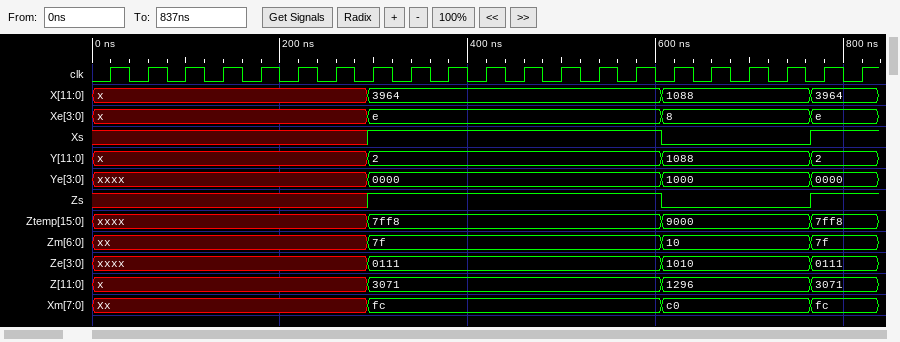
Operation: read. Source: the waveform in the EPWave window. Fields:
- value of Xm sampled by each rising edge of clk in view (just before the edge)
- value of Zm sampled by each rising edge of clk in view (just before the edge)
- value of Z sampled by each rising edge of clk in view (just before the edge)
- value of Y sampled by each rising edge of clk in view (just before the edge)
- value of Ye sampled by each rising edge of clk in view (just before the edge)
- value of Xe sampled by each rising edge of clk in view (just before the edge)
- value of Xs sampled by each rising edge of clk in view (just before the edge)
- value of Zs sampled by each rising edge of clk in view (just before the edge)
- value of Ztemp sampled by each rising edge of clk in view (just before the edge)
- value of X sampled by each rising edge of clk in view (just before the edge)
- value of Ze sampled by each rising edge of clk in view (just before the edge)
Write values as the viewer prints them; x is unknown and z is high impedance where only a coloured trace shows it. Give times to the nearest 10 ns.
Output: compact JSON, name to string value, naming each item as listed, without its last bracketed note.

{"value of Xm sampled by each rising edge of clk in view": "Xx, Xx, Xx, Xx, Xx, Xx, Xx, fc, fc, fc, fc, fc, fc, fc, fc, c0, c0, c0, c0, fc, fc", "value of Zm sampled by each rising edge of clk in view": "xx, xx, xx, xx, xx, xx, xx, 7f, 7f, 7f, 7f, 7f, 7f, 7f, 7f, 10, 10, 10, 10, 7f, 7f", "value of Z sampled by each rising edge of clk in view": "x, x, x, x, x, x, x, 3071, 3071, 3071, 3071, 3071, 3071, 3071, 3071, 1296, 1296, 1296, 1296, 3071, 3071", "value of Y sampled by each rising edge of clk in view": "x, x, x, x, x, x, x, 2, 2, 2, 2, 2, 2, 2, 2, 1088, 1088, 1088, 1088, 2, 2", "value of Ye sampled by each rising edge of clk in view": "xxxx, xxxx, xxxx, xxxx, xxxx, xxxx, xxxx, 0000, 0000, 0000, 0000, 0000, 0000, 0000, 0000, 1000, 1000, 1000, 1000, 0000, 0000", "value of Xe sampled by each rising edge of clk in view": "x, x, x, x, x, x, x, e, e, e, e, e, e, e, e, 8, 8, 8, 8, e, e", "value of Xs sampled by each rising edge of clk in view": "x x x x x x x 1 1 1 1 1 1 1 1 0 0 0 0 1 1", "value of Zs sampled by each rising edge of clk in view": "x x x x x x x 1 1 1 1 1 1 1 1 0 0 0 0 1 1", "value of Ztemp sampled by each rising edge of clk in view": "xxxx, xxxx, xxxx, xxxx, xxxx, xxxx, xxxx, 7ff8, 7ff8, 7ff8, 7ff8, 7ff8, 7ff8, 7ff8, 7ff8, 9000, 9000, 9000, 9000, 7ff8, 7ff8", "value of X sampled by each rising edge of clk in view": "x, x, x, x, x, x, x, 3964, 3964, 3964, 3964, 3964, 3964, 3964, 3964, 1088, 1088, 1088, 1088, 3964, 3964", "value of Ze sampled by each rising edge of clk in view": "xxxx, xxxx, xxxx, xxxx, xxxx, xxxx, xxxx, 0111, 0111, 0111, 0111, 0111, 0111, 0111, 0111, 1010, 1010, 1010, 1010, 0111, 0111"}
